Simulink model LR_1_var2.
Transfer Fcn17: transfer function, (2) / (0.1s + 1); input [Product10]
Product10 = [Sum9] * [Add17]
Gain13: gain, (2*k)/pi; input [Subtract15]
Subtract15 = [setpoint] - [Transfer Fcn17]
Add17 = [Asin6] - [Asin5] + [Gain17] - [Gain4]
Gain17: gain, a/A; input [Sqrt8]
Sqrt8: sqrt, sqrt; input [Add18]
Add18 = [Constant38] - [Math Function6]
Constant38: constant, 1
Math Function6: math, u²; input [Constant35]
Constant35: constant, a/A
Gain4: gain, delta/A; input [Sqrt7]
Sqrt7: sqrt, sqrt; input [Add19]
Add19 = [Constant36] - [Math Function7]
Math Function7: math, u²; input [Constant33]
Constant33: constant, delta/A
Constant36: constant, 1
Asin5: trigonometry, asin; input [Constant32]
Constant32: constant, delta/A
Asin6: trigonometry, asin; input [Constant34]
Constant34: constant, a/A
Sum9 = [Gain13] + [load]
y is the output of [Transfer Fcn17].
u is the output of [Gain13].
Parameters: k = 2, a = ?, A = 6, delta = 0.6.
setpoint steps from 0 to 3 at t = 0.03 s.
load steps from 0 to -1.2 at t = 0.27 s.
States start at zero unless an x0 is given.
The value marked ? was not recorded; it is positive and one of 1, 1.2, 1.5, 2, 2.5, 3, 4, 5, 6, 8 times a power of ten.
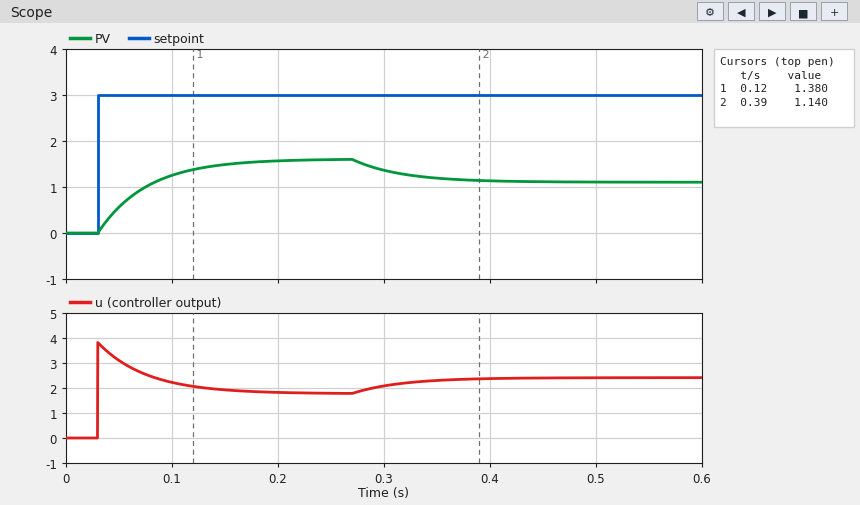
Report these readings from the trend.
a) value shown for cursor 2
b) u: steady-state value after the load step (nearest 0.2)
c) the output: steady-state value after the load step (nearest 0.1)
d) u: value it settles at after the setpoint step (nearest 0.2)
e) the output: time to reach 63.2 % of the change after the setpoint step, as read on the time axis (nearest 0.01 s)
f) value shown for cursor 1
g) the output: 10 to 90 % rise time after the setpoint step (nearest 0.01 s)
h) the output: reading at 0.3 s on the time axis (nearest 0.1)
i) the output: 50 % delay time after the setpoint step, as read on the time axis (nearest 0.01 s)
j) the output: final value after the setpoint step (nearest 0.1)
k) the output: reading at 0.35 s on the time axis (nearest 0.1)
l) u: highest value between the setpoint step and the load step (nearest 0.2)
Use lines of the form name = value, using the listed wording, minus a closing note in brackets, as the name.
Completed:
value shown for cursor 2 = 1.140
u: steady-state value after the load step = 2.4
the output: steady-state value after the load step = 1.1
u: value it settles at after the setpoint step = 1.8
the output: time to reach 63.2 % of the change after the setpoint step, as read on the time axis = 0.08 s
value shown for cursor 1 = 1.380
the output: 10 to 90 % rise time after the setpoint step = 0.10 s
the output: reading at 0.3 s on the time axis = 1.4
the output: 50 % delay time after the setpoint step, as read on the time axis = 0.06 s
the output: final value after the setpoint step = 1.6
the output: reading at 0.35 s on the time axis = 1.2
u: highest value between the setpoint step and the load step = 3.8
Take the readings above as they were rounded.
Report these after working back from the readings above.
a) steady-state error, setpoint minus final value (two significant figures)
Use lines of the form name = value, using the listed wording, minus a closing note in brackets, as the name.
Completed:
steady-state error, setpoint minus final value = 1.4
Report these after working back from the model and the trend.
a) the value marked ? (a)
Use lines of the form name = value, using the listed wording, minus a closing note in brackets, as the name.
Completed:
the value marked ? = 2
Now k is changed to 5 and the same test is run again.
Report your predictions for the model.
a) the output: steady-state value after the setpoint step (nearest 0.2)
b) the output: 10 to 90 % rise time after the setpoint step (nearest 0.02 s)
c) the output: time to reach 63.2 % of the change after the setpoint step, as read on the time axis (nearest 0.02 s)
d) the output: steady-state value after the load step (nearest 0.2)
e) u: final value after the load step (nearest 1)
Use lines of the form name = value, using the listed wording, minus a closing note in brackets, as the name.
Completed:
the output: steady-state value after the setpoint step = 2.2
the output: 10 to 90 % rise time after the setpoint step = 0.06 s
the output: time to reach 63.2 % of the change after the setpoint step, as read on the time axis = 0.06 s
the output: steady-state value after the load step = 2.0
u: final value after the load step = 3
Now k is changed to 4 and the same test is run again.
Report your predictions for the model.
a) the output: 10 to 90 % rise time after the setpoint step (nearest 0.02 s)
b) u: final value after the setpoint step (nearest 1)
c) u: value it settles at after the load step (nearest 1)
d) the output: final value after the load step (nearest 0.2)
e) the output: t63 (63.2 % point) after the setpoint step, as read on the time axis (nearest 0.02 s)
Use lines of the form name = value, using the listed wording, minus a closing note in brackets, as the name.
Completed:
the output: 10 to 90 % rise time after the setpoint step = 0.06 s
u: final value after the setpoint step = 2
u: value it settles at after the load step = 3
the output: final value after the load step = 1.8
the output: t63 (63.2 % point) after the setpoint step, as read on the time axis = 0.06 s
